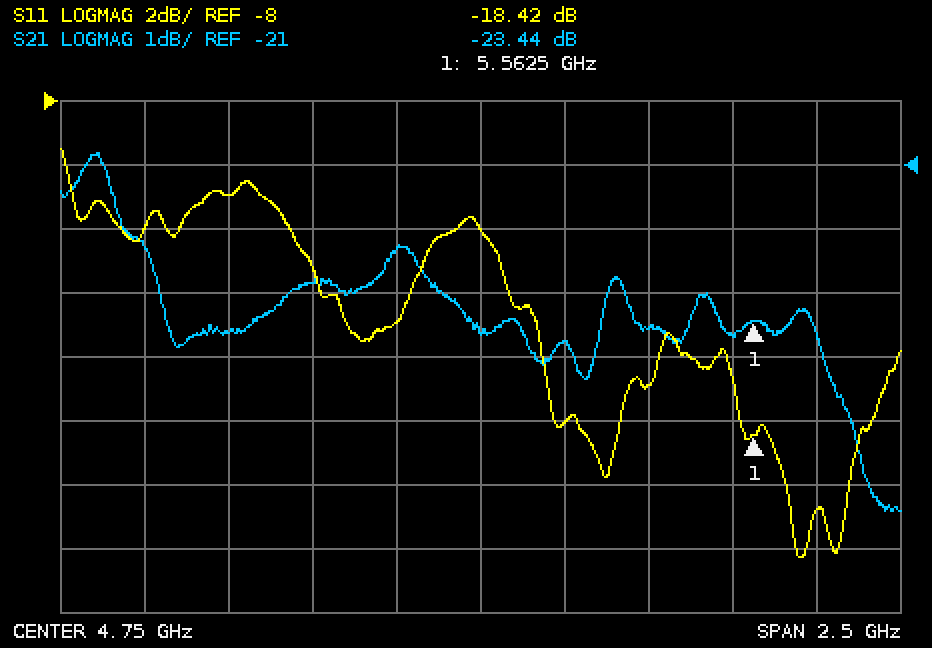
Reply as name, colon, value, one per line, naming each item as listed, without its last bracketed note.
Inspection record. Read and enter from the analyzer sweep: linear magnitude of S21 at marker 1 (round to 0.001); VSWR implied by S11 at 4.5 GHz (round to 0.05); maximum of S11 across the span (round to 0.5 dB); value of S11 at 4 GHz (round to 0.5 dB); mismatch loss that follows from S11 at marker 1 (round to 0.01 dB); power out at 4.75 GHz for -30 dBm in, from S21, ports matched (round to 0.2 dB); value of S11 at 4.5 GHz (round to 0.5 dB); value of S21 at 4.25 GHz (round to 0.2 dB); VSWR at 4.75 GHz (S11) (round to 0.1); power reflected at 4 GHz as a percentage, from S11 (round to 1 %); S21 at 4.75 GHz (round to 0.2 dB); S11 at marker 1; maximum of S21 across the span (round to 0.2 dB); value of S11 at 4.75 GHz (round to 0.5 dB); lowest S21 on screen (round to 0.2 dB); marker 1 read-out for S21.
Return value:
linear magnitude of S21 at marker 1: 0.067
VSWR implied by S11 at 4.5 GHz: 1.45
maximum of S11 across the span: -9.5 dB
value of S11 at 4 GHz: -11.0 dB
mismatch loss that follows from S11 at marker 1: 0.06 dB
power out at 4.75 GHz for -30 dBm in, from S21, ports matched: -53.6 dBm
value of S11 at 4.5 GHz: -15.0 dB
value of S21 at 4.25 GHz: -22.8 dB
VSWR at 4.75 GHz (S11): 1.7
power reflected at 4 GHz as a percentage, from S11: 8 %
S21 at 4.75 GHz: -23.6 dB
S11 at marker 1: -18.42 dB
maximum of S21 across the span: -20.8 dB
value of S11 at 4.75 GHz: -12.0 dB
lowest S21 on screen: -26.4 dB
marker 1 read-out for S21: -23.44 dB
